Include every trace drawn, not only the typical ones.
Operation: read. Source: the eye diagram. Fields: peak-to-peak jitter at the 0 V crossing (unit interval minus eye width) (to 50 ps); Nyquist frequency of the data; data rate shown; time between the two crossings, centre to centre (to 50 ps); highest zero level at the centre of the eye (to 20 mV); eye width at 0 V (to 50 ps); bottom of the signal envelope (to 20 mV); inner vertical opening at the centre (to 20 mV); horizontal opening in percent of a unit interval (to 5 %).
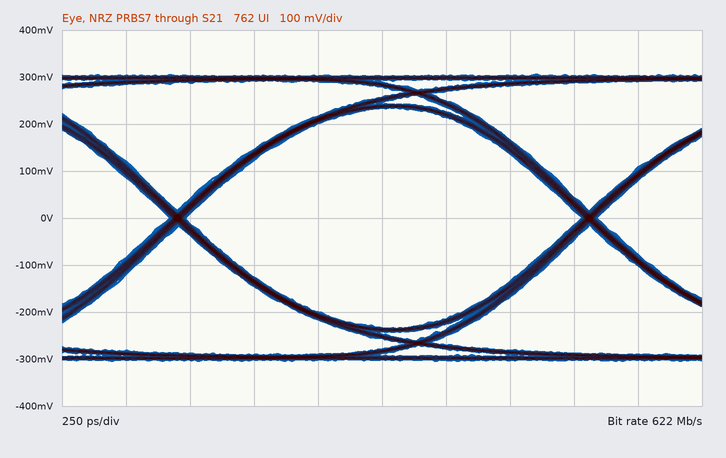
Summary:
50 ps
311 MHz
622 Mb/s
1.60 ns
-240 mV
1.55 ns
-300 mV
460 mV
95 %
